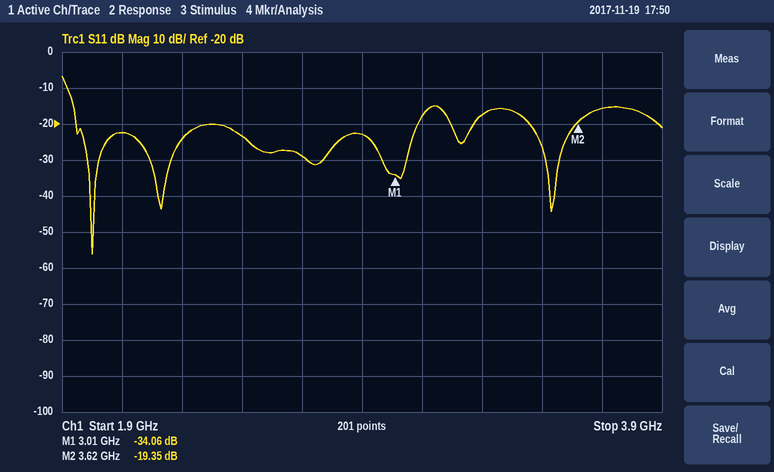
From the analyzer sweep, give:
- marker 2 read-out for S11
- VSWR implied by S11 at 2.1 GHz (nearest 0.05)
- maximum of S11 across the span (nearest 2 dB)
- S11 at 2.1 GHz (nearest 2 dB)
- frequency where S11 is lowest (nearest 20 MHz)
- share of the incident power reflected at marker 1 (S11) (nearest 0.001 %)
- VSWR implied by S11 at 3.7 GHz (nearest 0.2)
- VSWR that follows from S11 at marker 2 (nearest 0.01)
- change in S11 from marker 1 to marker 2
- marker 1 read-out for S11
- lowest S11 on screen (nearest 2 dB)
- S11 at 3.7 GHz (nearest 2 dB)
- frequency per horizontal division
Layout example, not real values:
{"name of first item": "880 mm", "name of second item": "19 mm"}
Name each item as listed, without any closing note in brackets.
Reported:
{"marker 2 read-out for S11": "-19.35 dB", "VSWR implied by S11 at 2.1 GHz": "1.15", "maximum of S11 across the span": "-6 dB", "S11 at 2.1 GHz": "-22 dB", "frequency where S11 is lowest": "2.00 GHz", "share of the incident power reflected at marker 1 (S11)": "0.039 %", "VSWR implied by S11 at 3.7 GHz": "1.4", "VSWR that follows from S11 at marker 2": "1.24", "change in S11 from marker 1 to marker 2": "14.71 dB", "marker 1 read-out for S11": "-34.06 dB", "lowest S11 on screen": "-56 dB", "S11 at 3.7 GHz": "-16 dB", "frequency per horizontal division": "200 MHz"}
